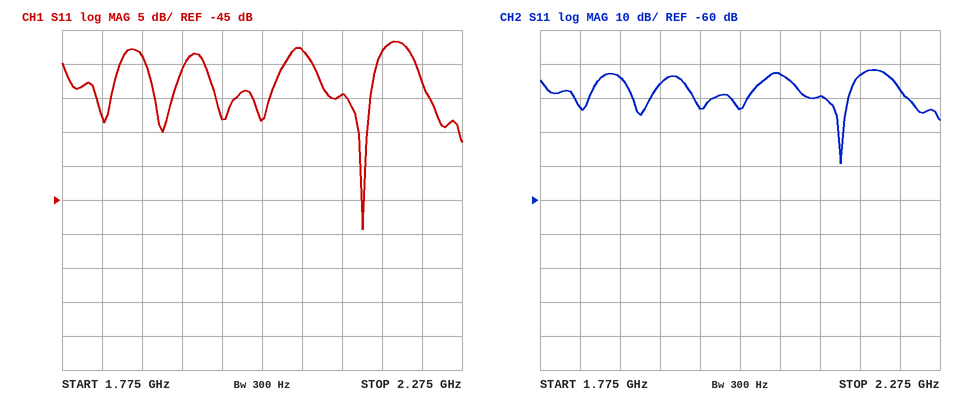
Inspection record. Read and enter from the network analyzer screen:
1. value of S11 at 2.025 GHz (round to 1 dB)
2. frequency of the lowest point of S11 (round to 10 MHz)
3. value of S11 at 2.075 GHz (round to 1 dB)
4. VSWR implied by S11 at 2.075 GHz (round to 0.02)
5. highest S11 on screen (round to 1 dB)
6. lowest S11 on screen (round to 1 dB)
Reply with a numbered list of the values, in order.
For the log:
1. -33 dB
2. 2.15 GHz
3. -23 dB
4. 1.16
5. -22 dB
6. -49 dB
